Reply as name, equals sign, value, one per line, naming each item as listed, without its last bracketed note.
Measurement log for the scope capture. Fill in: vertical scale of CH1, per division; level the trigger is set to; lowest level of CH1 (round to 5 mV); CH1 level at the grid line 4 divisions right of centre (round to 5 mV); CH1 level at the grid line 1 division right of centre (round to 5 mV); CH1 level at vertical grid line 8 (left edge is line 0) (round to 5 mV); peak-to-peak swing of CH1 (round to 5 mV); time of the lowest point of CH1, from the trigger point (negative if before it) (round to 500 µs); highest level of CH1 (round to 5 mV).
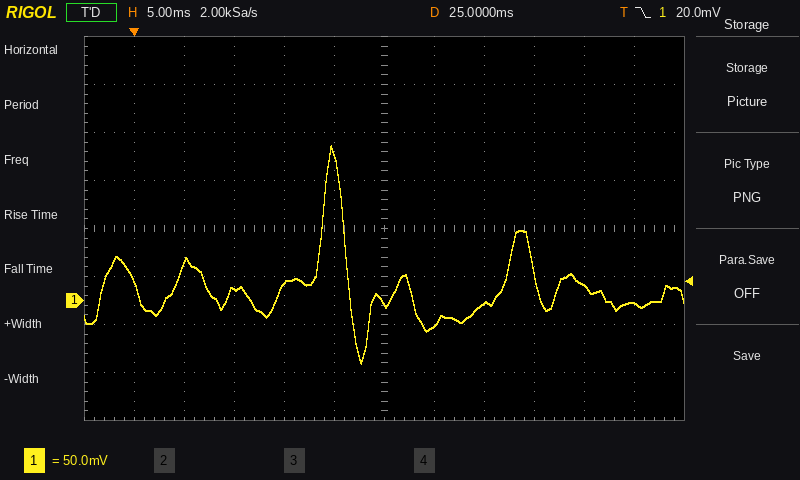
vertical scale of CH1, per division = 50 mV
level the trigger is set to = 20.0 mV
lowest level of CH1 = -65 mV
CH1 level at the grid line 4 divisions right of centre = 15 mV
CH1 level at the grid line 1 division right of centre = -25 mV
CH1 level at vertical grid line 8 (left edge is line 0) = -5 mV
peak-to-peak swing of CH1 = 225 mV
time of the lowest point of CH1, from the trigger point (negative if before it) = +22.5 ms
highest level of CH1 = 160 mV
